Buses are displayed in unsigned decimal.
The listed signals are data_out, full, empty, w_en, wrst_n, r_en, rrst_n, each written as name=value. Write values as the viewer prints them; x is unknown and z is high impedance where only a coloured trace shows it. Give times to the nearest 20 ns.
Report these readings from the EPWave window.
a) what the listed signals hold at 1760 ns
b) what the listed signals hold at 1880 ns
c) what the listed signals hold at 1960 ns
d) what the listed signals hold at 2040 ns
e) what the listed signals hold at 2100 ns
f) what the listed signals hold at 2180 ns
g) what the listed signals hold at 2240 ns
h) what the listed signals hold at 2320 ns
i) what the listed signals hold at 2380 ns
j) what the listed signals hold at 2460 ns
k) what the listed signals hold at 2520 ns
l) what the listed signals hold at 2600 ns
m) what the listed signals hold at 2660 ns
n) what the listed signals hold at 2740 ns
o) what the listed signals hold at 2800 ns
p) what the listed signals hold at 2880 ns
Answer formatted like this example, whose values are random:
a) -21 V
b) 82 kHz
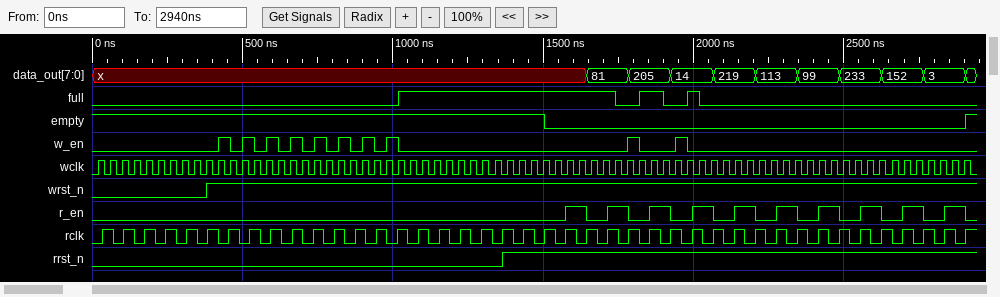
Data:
a) data_out=81, full=0, empty=0, w_en=0, wrst_n=1, r_en=1, rrst_n=1
b) data_out=205, full=1, empty=0, w_en=0, wrst_n=1, r_en=1, rrst_n=1
c) data_out=14, full=0, empty=0, w_en=1, wrst_n=1, r_en=0, rrst_n=1
d) data_out=14, full=0, empty=0, w_en=0, wrst_n=1, r_en=1, rrst_n=1
e) data_out=219, full=0, empty=0, w_en=0, wrst_n=1, r_en=0, rrst_n=1
f) data_out=219, full=0, empty=0, w_en=0, wrst_n=1, r_en=1, rrst_n=1
g) data_out=113, full=0, empty=0, w_en=0, wrst_n=1, r_en=0, rrst_n=1
h) data_out=113, full=0, empty=0, w_en=0, wrst_n=1, r_en=1, rrst_n=1
i) data_out=99, full=0, empty=0, w_en=0, wrst_n=1, r_en=0, rrst_n=1
j) data_out=99, full=0, empty=0, w_en=0, wrst_n=1, r_en=1, rrst_n=1
k) data_out=233, full=0, empty=0, w_en=0, wrst_n=1, r_en=0, rrst_n=1
l) data_out=233, full=0, empty=0, w_en=0, wrst_n=1, r_en=1, rrst_n=1
m) data_out=152, full=0, empty=0, w_en=0, wrst_n=1, r_en=0, rrst_n=1
n) data_out=152, full=0, empty=0, w_en=0, wrst_n=1, r_en=1, rrst_n=1
o) data_out=3, full=0, empty=0, w_en=0, wrst_n=1, r_en=0, rrst_n=1
p) data_out=3, full=0, empty=0, w_en=0, wrst_n=1, r_en=1, rrst_n=1
